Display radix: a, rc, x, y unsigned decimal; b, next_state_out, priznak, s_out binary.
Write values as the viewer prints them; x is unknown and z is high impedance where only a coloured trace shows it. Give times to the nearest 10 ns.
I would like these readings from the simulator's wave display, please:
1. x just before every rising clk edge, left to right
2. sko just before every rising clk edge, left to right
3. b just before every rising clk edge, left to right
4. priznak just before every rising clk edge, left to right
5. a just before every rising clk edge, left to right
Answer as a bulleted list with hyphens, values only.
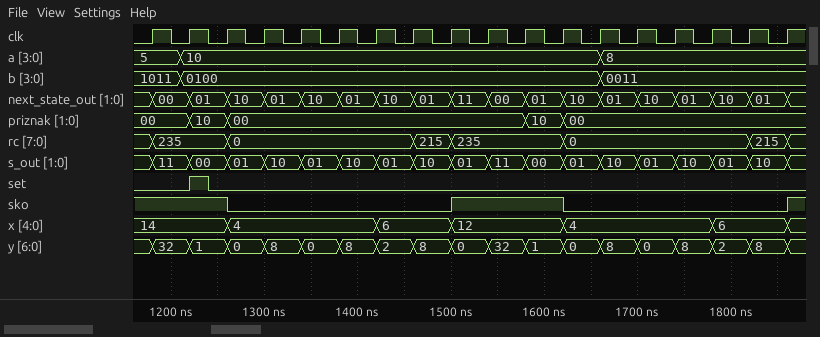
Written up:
- 14, 14, 14, 4, 4, 4, 4, 6, 6, 12, 12, 12, 4, 4, 4, 4, 6, 6
- 1 1 1 0 0 0 0 0 0 1 1 1 0 0 0 0 0 0
- 1011, 0100, 0100, 0100, 0100, 0100, 0100, 0100, 0100, 0100, 0100, 0100, 0100, 0011, 0011, 0011, 0011, 0011
- 00, 00, 10, 00, 00, 00, 00, 00, 00, 00, 00, 10, 00, 00, 00, 00, 00, 00
- 5, 10, 10, 10, 10, 10, 10, 10, 10, 10, 10, 10, 10, 8, 8, 8, 8, 8
